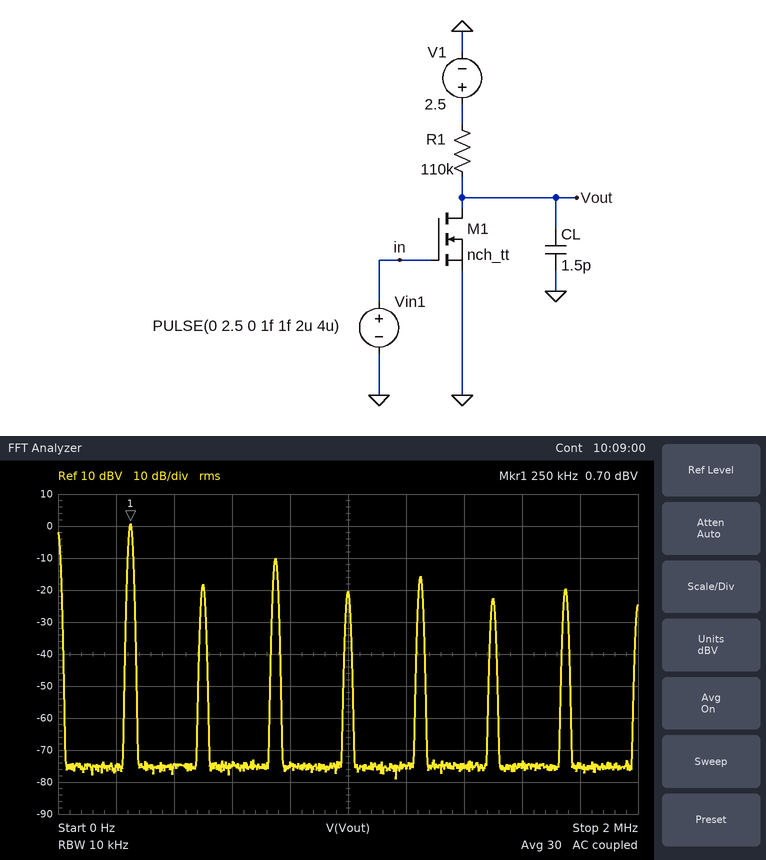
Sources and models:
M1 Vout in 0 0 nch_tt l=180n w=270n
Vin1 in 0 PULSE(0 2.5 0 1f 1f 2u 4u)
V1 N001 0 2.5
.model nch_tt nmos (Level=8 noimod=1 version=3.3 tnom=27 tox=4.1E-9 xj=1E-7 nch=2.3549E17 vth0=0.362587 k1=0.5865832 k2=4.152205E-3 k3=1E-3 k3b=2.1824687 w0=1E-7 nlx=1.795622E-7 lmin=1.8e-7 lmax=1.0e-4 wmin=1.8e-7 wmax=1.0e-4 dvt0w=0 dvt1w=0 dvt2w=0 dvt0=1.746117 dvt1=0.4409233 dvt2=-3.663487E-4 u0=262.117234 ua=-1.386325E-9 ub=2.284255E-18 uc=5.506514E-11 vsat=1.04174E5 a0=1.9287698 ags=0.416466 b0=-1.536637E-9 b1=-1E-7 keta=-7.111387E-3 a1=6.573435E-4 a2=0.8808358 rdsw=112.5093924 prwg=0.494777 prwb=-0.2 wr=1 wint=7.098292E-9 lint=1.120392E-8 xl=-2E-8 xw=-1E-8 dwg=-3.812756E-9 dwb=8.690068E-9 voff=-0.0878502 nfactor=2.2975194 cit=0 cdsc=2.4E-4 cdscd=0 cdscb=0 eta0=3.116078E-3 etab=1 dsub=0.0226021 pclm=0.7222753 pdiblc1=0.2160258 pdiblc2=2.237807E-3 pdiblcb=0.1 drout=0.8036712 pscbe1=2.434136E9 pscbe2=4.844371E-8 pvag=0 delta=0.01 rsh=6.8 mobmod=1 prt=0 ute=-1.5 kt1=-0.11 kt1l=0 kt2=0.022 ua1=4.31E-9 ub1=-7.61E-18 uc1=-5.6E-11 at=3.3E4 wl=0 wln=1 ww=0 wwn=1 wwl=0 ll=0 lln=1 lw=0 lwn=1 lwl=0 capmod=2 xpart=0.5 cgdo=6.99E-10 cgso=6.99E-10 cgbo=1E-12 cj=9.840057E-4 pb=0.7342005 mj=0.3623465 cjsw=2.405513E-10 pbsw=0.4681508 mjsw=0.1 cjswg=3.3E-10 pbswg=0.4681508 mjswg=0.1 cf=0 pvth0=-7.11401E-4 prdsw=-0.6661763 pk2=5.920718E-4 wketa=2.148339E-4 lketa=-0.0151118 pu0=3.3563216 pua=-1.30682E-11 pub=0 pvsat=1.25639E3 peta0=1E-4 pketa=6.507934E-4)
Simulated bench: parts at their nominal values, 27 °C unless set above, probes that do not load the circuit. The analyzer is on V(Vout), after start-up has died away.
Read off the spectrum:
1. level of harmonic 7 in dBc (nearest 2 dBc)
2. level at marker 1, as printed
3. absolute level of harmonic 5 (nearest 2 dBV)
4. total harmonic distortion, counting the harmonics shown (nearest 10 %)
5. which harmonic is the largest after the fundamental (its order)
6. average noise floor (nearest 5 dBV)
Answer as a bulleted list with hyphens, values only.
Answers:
- -20 dBc
- 0.70 dBV
- -16 dBV
- 40 %
- 3
- -75 dBV
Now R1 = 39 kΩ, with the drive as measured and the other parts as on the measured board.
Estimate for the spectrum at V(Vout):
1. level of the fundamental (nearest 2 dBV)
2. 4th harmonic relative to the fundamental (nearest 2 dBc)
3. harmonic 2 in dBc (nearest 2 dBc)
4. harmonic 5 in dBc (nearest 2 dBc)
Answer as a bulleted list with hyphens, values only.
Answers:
- 0 dBV
- -28 dBc
- -28 dBc
- -14 dBc
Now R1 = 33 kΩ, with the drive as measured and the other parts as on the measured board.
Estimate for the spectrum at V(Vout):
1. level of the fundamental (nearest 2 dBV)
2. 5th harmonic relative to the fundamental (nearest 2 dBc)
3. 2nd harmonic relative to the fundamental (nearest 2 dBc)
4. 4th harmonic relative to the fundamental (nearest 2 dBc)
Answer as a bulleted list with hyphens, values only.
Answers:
- 0 dBV
- -14 dBc
- -30 dBc
- -30 dBc
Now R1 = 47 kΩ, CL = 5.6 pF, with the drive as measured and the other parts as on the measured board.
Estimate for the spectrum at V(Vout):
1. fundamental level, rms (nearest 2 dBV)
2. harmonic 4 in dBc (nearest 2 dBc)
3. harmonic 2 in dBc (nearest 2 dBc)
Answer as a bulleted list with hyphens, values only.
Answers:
- 0 dBV
- -20 dBc
- -16 dBc
